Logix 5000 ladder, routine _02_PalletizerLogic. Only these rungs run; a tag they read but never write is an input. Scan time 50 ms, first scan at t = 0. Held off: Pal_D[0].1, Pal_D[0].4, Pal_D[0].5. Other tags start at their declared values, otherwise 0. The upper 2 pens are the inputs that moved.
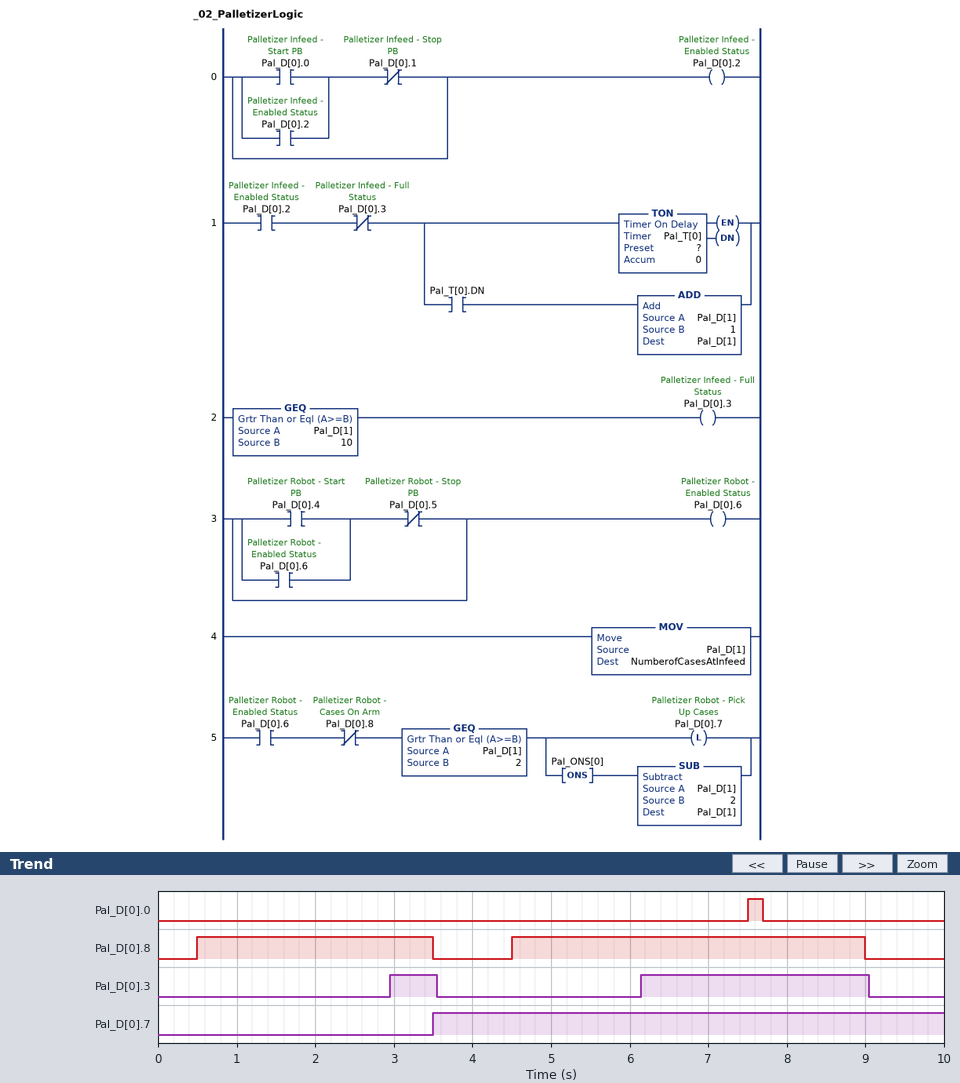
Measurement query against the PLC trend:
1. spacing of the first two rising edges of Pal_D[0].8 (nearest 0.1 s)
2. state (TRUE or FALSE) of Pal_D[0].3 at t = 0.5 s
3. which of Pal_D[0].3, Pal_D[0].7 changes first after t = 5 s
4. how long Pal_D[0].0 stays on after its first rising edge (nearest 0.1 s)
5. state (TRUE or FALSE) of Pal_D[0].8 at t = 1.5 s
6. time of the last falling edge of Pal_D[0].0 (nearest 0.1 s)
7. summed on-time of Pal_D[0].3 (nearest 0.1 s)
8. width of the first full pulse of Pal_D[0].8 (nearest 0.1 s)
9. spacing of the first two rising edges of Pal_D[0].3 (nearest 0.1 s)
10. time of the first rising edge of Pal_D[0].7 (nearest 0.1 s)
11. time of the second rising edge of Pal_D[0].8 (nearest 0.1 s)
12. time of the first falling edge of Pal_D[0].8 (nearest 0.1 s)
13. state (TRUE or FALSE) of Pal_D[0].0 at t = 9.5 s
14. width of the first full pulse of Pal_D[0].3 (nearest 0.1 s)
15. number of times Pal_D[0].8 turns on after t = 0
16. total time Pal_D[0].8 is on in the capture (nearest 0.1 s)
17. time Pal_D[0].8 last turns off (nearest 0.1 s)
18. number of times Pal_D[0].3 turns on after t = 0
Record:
4.0 s
FALSE
Pal_D[0].3
0.2 s
TRUE
7.7 s
3.5 s
3.0 s
3.2 s
3.5 s
4.5 s
3.5 s
FALSE
0.6 s
2
7.5 s
9.0 s
2
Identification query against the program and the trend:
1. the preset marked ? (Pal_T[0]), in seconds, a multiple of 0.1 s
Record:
2.5 s
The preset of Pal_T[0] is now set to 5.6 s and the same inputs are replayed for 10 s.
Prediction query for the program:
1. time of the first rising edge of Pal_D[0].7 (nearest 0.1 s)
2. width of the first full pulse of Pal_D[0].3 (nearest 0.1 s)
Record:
9.0 s
3.0 s
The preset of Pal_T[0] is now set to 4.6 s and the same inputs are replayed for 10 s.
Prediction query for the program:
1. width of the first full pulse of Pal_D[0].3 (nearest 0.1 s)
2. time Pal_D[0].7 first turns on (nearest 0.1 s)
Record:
4.0 s
9.0 s
